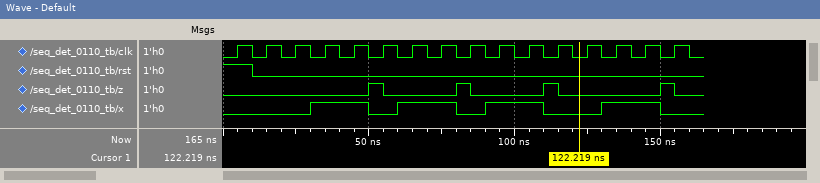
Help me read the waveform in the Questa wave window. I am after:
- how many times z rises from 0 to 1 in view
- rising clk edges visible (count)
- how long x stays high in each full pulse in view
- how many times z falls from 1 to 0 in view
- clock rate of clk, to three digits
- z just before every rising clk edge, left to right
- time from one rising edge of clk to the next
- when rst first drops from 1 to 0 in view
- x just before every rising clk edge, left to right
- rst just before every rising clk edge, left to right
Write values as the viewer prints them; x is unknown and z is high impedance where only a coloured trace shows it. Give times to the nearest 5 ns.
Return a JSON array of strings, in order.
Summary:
["4", "16", "20 ns, 20 ns, 20 ns, 20 ns", "4", "100 MHz", "0 0 0 0 0 1 0 0 1 0 0 1 0 0 0 1", "10 ns", "10 ns", "0 0 0 1 1 0 1 1 0 1 1 0 0 1 1 0", "1 0 0 0 0 0 0 0 0 0 0 0 0 0 0 0"]
